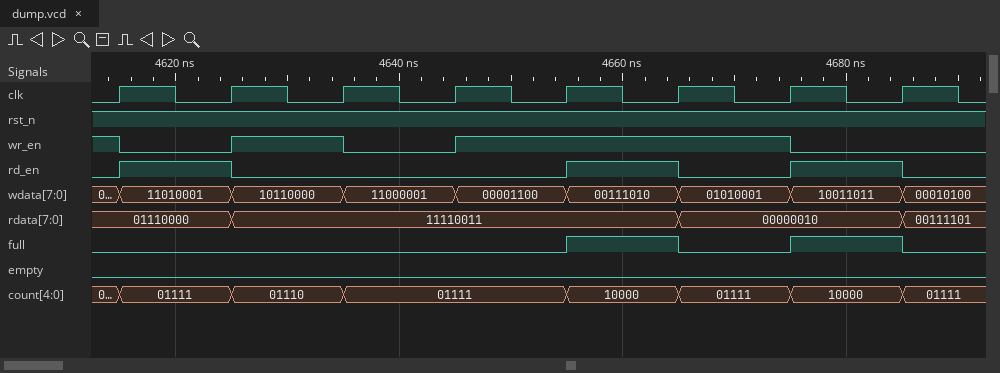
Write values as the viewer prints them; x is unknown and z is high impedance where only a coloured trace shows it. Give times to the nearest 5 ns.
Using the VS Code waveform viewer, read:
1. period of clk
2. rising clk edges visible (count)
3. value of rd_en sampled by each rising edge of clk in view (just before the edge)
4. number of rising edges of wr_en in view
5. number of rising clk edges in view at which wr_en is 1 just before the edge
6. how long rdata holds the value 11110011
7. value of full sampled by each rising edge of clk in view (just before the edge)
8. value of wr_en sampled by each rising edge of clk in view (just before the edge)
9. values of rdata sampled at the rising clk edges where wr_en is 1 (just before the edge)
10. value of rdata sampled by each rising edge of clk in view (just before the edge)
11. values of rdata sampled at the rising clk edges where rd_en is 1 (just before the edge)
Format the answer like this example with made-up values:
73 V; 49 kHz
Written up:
10 ns; 8; 0 1 0 0 0 1 0 1; 2; 5; 40 ns; 0 0 0 0 0 1 0 1; 1 0 1 0 1 1 1 0; 01110000, 11110011, 11110011, 11110011, 00000010; 01110000, 01110000, 11110011, 11110011, 11110011, 11110011, 00000010, 00000010; 01110000, 11110011, 00000010
